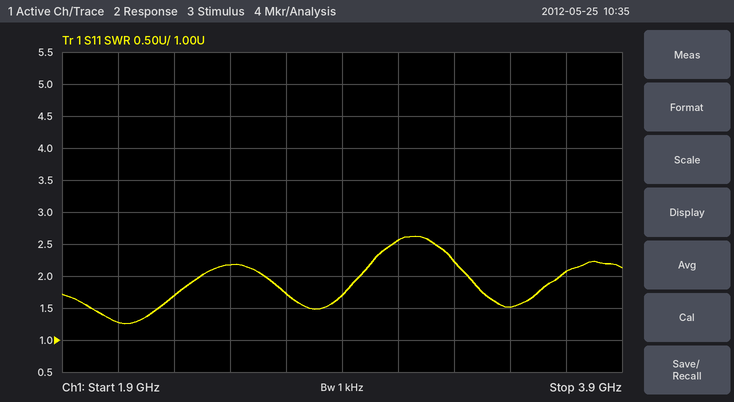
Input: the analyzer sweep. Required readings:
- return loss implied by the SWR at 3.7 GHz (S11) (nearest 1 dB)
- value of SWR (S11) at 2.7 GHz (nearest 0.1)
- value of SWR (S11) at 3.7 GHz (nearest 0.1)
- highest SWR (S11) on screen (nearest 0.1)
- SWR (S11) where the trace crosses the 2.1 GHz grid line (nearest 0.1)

9 dB
1.7
2.1
2.6
1.3
